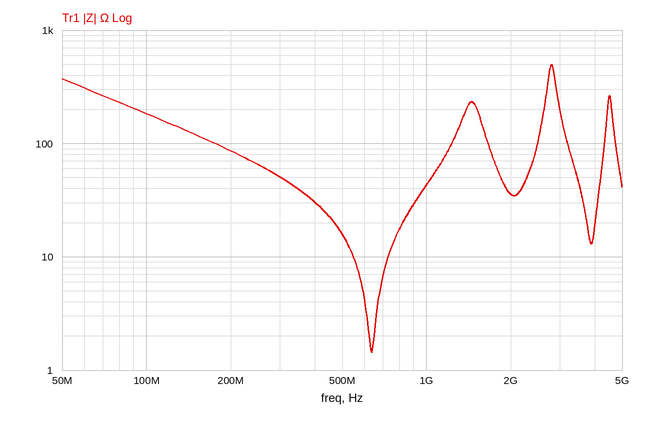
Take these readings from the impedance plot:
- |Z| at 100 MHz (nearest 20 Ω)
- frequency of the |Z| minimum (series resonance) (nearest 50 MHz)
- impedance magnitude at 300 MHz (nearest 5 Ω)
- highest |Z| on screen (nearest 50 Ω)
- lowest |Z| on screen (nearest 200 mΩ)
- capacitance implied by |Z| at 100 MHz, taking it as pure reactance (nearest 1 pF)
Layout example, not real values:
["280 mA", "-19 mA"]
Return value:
["180 Ω", "650 MHz", "50 Ω", "500 Ω", "1.4 Ω", "9 pF"]
